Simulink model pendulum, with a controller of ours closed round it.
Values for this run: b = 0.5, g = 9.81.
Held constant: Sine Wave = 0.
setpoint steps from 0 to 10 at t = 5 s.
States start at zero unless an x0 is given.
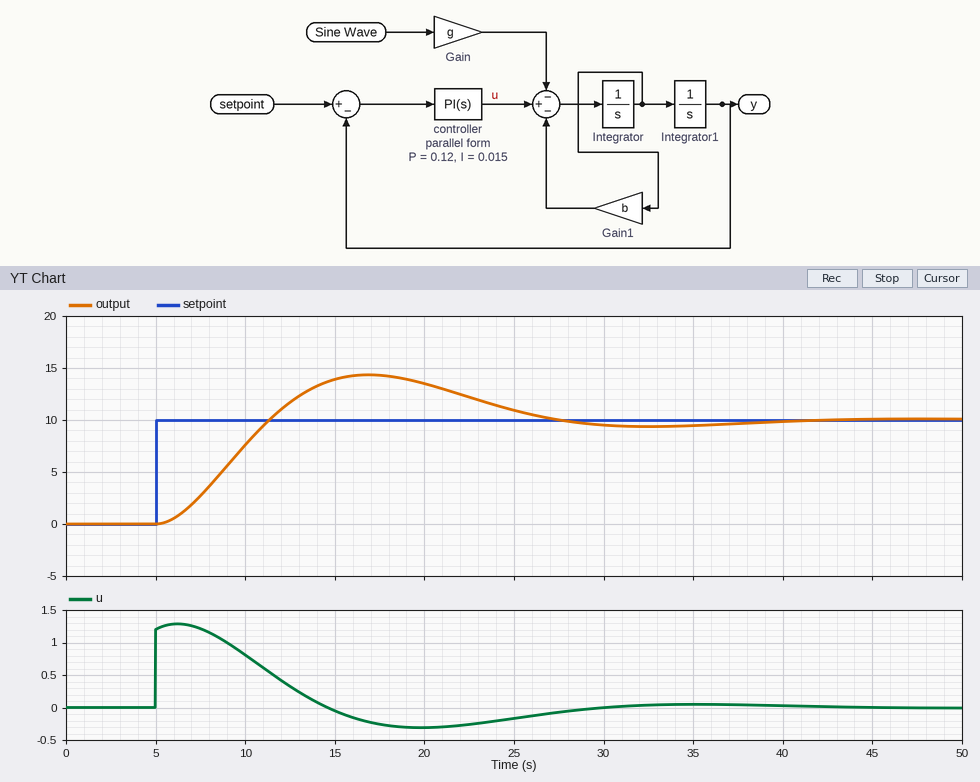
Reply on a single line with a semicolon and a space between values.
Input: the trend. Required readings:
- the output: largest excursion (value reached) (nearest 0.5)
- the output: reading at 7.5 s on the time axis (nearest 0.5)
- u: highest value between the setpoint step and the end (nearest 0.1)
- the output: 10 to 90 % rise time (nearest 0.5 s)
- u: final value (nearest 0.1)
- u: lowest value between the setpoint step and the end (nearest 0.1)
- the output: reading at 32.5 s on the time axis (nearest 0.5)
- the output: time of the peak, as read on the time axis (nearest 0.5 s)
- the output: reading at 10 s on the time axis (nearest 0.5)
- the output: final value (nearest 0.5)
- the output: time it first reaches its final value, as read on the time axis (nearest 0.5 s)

14.5; 2.5; 1.3; 4.5 s; 0.0; -0.3; 9.5; 17.0 s; 7.5; 10.0; 11.5 s
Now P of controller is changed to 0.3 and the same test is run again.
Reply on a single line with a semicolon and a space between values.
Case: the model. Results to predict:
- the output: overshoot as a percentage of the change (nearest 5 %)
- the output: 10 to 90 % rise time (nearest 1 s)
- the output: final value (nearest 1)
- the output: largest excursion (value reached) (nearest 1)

30 %; 3 s; 10; 13
